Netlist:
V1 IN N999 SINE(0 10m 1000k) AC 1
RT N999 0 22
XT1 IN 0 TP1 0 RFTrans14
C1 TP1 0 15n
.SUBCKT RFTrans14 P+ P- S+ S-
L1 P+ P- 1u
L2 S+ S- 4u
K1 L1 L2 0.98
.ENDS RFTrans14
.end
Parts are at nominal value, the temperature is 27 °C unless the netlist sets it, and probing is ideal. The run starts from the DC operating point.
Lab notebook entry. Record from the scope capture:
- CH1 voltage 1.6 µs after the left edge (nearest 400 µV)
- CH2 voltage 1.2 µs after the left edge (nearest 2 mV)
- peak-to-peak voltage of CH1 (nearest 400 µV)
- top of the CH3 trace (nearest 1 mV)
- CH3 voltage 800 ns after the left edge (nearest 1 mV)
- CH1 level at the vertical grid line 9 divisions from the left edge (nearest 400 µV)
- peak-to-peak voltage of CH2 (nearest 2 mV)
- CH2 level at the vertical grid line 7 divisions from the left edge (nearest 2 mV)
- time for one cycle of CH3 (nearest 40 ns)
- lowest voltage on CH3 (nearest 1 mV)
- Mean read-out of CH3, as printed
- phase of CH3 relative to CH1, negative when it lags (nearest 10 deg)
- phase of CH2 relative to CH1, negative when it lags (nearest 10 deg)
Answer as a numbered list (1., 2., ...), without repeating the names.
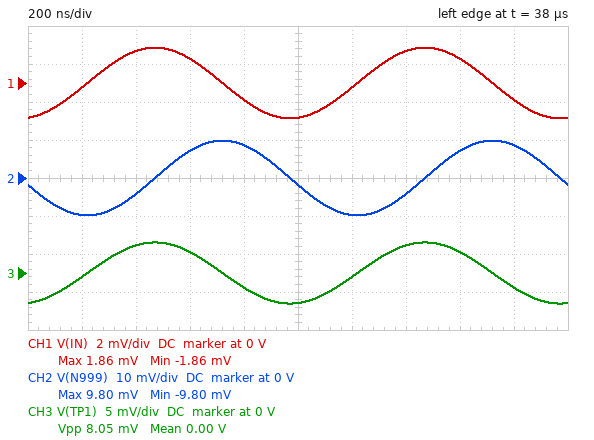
1. 1.2 mV
2. -10 mV
3. 3.6 mV
4. 4 mV
5. -2 mV
6. -800 µV
7. 20 mV
8. -4 mV
9. 1.00 µs
10. -4 mV
11. 0.00 V
12. 0 deg
13. -90 deg
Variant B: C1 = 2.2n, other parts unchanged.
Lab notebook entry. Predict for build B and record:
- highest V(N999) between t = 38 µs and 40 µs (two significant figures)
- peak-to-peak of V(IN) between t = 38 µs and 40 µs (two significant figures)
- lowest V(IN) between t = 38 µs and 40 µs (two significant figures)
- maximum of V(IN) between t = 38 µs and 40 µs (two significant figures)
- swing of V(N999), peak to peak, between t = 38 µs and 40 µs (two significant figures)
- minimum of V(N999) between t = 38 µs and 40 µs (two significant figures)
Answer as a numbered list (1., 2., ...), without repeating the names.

1. 9.2 mV
2. 7.9 mV
3. -4.0 mV
4. 4.0 mV
5. 18 mV
6. -9.2 mV
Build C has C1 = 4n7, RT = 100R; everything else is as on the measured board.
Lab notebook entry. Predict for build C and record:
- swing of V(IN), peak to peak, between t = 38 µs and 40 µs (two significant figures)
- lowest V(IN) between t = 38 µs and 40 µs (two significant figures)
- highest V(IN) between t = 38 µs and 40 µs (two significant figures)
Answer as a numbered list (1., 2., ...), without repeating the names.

1. 4.6 mV
2. -2.3 mV
3. 2.3 mV
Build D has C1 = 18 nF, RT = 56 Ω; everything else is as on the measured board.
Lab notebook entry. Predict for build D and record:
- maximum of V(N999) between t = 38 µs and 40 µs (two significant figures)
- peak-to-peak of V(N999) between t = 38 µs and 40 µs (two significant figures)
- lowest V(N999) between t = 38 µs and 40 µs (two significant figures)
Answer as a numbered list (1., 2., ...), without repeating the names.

1. 10 mV
2. 20 mV
3. -10 mV
